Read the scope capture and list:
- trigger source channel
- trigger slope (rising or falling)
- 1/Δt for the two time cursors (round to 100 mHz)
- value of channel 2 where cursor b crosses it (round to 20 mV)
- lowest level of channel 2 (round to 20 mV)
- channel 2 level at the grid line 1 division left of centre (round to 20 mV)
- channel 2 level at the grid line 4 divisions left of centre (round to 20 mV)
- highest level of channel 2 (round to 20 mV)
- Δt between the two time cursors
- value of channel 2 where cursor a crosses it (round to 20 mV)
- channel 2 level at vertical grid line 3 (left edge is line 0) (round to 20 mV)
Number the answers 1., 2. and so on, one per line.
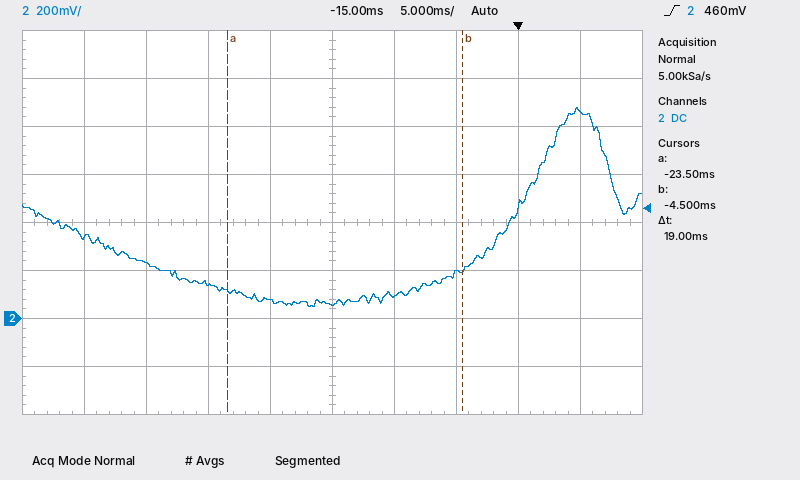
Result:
1. channel 2
2. rising
3. 52.6 Hz
4. 200 mV
5. 40 mV
6. 80 mV
7. 340 mV
8. 880 mV
9. 19 ms
10. 120 mV
11. 140 mV
